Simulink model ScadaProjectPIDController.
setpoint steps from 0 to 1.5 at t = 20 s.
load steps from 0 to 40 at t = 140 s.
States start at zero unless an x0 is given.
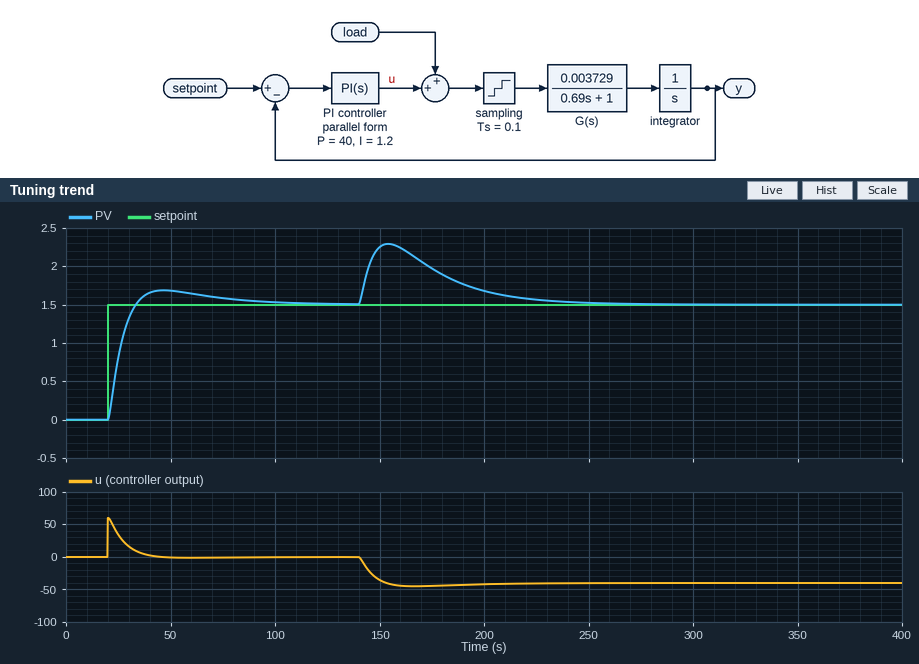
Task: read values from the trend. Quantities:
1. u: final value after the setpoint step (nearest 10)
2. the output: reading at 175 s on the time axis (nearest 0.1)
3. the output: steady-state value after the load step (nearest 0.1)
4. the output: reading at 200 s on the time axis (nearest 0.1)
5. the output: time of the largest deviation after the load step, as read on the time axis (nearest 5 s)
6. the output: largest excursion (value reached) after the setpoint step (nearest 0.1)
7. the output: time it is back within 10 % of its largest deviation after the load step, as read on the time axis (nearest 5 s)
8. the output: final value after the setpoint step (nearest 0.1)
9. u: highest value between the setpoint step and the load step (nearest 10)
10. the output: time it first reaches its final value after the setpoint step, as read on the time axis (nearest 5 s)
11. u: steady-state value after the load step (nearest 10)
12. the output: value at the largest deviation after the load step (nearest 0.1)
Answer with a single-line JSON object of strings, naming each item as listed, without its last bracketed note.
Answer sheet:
{"u: final value after the setpoint step": "0", "the output: reading at 175 s on the time axis": "2.0", "the output: steady-state value after the load step": "1.5", "the output: reading at 200 s on the time axis": "1.7", "the output: time of the largest deviation after the load step, as read on the time axis": "155 s", "the output: largest excursion (value reached) after the setpoint step": "1.7", "the output: time it is back within 10 % of its largest deviation after the load step, as read on the time axis": "220 s", "the output: final value after the setpoint step": "1.5", "u: highest value between the setpoint step and the load step": "60", "the output: time it first reaches its final value after the setpoint step, as read on the time axis": "35 s", "u: steady-state value after the load step": "-40", "the output: value at the largest deviation after the load step": "2.3"}
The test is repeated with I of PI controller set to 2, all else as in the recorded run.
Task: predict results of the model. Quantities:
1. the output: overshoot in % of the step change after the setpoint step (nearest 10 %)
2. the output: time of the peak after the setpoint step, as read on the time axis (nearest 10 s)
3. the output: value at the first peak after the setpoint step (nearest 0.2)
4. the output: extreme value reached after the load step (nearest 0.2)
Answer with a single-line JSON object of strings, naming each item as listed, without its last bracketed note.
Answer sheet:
{"the output: overshoot in % of the step change after the setpoint step": "20 %", "the output: time of the peak after the setpoint step, as read on the time axis": "40 s", "the output: value at the first peak after the setpoint step": "1.8", "the output: extreme value reached after the load step": "2.2"}
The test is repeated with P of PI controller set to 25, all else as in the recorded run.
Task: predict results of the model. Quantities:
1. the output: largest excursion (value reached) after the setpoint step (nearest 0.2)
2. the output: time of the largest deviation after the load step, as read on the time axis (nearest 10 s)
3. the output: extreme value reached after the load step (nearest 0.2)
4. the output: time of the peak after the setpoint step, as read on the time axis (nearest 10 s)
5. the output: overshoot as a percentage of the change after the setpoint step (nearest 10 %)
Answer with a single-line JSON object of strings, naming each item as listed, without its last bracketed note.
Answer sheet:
{"the output: largest excursion (value reached) after the setpoint step": "1.8", "the output: time of the largest deviation after the load step, as read on the time axis": "160 s", "the output: extreme value reached after the load step": "2.6", "the output: time of the peak after the setpoint step, as read on the time axis": "50 s", "the output: overshoot as a percentage of the change after the setpoint step": "20 %"}
